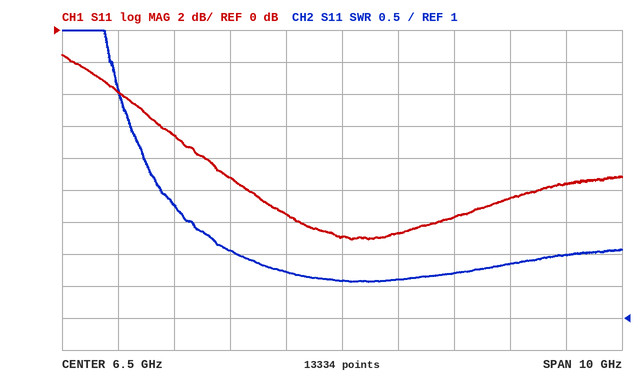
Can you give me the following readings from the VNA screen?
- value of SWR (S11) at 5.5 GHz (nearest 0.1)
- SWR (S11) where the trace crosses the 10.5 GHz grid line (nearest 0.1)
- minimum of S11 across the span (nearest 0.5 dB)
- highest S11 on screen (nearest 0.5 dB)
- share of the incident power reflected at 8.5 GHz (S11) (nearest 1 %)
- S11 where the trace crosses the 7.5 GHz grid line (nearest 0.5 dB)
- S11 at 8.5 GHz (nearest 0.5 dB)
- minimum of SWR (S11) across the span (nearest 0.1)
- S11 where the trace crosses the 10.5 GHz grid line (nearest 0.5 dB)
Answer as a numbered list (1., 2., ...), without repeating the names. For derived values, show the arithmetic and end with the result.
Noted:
1. 1.7
2. 2.0
3. -13.0 dB
4. -1.5 dB
5. 10^(-11.5/10) ≈ 7 %
6. -12.5 dB
7. -11.5 dB
8. 1.6
9. -9.5 dB
